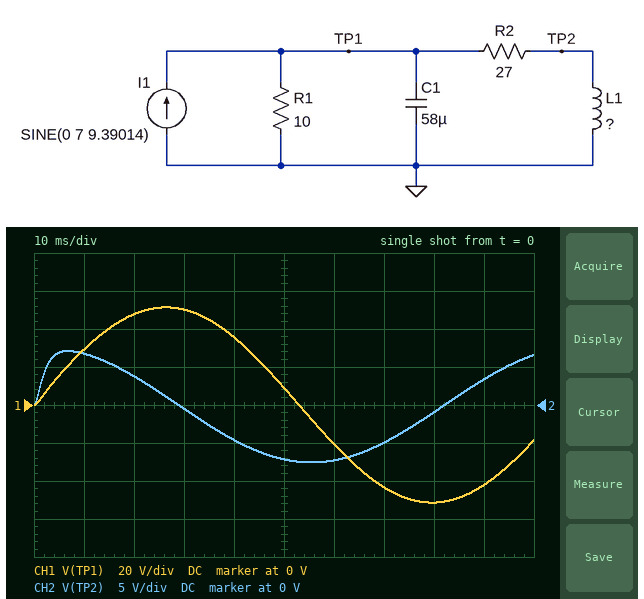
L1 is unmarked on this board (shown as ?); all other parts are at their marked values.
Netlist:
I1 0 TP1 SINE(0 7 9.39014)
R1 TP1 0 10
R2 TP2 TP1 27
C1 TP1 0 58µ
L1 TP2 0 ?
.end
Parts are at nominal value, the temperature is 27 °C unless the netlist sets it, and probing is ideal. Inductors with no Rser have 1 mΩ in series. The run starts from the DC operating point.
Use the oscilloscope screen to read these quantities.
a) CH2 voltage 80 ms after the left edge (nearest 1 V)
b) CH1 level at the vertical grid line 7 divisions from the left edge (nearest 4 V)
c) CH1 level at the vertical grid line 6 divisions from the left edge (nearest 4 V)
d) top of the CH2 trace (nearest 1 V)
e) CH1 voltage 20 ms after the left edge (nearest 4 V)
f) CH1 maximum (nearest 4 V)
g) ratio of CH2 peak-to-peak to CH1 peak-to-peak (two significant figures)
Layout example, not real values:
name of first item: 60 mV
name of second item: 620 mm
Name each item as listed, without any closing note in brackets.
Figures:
CH2 voltage 80 ms after the left edge: -1 V
CH1 level at the vertical grid line 7 divisions from the left edge: -44 V
CH1 level at the vertical grid line 6 divisions from the left edge: -20 V
top of the CH2 trace: 7 V
CH1 voltage 20 ms after the left edge: 48 V
CH1 maximum: 52 V
ratio of CH2 peak-to-peak to CH1 peak-to-peak: 0.14
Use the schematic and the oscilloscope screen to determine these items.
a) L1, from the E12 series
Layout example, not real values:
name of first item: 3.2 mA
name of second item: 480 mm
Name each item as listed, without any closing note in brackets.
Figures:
L1, from the E12 series: 68 mH
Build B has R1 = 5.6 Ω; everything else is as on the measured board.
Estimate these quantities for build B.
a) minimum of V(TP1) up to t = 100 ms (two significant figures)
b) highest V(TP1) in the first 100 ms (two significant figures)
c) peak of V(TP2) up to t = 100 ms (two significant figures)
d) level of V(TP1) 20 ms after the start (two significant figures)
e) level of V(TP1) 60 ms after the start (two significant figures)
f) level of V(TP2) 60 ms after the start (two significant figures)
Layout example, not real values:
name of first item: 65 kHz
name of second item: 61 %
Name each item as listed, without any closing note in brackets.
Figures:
minimum of V(TP1) up to t = 100 ms: -33 V
highest V(TP1) in the first 100 ms: 33 V
peak of V(TP2) up to t = 100 ms: 4.4 V
level of V(TP1) 20 ms after the start: 30 V
level of V(TP1) 60 ms after the start: -13 V
level of V(TP2) 60 ms after the start: -4.6 V
